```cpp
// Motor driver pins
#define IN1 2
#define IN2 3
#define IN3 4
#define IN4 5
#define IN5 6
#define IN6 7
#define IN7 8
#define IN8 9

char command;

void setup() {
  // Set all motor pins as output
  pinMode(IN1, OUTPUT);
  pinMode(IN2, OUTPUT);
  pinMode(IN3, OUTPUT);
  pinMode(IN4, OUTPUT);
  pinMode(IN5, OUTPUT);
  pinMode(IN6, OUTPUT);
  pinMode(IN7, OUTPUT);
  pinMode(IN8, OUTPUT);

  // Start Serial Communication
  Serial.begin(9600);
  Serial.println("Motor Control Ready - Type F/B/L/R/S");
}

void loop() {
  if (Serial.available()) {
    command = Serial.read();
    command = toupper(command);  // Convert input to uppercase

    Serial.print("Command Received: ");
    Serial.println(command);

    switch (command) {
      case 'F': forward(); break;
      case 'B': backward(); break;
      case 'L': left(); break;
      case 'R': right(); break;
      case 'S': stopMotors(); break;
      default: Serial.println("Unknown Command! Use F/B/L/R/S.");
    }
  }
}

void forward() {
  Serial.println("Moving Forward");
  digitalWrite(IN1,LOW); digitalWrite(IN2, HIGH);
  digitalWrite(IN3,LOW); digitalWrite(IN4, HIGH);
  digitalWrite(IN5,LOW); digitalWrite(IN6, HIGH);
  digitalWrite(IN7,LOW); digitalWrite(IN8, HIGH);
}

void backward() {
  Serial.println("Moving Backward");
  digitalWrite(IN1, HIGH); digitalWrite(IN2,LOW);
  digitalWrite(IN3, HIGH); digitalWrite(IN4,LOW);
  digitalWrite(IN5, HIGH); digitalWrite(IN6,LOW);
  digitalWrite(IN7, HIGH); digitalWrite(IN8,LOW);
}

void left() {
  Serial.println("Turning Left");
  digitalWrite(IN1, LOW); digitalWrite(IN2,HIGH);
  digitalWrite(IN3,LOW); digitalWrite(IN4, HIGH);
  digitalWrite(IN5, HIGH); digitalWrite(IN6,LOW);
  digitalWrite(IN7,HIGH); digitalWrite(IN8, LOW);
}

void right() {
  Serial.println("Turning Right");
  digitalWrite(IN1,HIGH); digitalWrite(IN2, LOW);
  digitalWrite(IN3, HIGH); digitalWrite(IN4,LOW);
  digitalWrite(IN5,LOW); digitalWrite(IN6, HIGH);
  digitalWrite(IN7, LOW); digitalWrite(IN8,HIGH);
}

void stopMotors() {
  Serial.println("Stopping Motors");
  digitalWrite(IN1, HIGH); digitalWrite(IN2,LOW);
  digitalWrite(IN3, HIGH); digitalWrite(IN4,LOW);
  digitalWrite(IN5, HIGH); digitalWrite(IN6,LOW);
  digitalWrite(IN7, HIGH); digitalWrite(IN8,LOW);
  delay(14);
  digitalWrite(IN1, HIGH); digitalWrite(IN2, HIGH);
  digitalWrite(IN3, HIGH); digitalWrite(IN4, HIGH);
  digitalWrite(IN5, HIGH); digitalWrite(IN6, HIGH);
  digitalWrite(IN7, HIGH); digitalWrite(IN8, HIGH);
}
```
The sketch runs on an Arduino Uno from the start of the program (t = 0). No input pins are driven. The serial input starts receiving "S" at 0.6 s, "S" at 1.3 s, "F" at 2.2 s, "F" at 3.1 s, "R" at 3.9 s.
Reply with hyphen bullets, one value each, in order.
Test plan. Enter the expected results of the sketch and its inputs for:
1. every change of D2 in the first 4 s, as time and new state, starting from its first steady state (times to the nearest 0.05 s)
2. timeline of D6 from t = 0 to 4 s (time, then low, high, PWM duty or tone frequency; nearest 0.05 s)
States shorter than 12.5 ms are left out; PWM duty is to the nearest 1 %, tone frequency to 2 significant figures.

- 0 s low; 0.6 s high; 2.2 s low; 3.9 s high
- 0 s low; 0.6 s high; 2.2 s low
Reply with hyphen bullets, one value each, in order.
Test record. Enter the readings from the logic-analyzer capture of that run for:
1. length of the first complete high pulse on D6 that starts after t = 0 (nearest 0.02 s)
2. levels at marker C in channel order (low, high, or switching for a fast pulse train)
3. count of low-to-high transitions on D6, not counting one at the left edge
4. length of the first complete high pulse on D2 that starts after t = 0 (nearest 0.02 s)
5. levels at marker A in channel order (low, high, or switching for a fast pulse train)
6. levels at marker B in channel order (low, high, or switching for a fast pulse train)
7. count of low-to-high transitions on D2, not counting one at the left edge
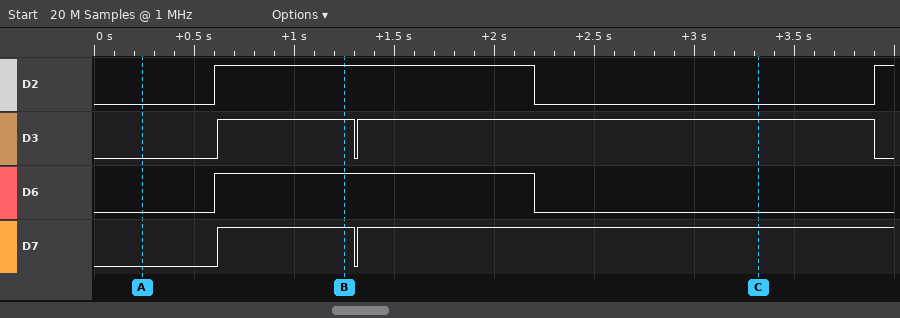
- 1.60 s
- D2 low, D3 high, D6 low, D7 high
- 1
- 1.60 s
- D2 low, D3 low, D6 low, D7 low
- D2 high, D3 high, D6 high, D7 high
- 2
